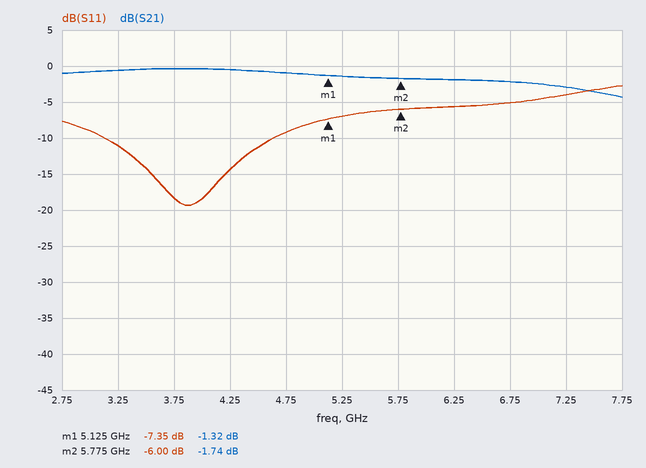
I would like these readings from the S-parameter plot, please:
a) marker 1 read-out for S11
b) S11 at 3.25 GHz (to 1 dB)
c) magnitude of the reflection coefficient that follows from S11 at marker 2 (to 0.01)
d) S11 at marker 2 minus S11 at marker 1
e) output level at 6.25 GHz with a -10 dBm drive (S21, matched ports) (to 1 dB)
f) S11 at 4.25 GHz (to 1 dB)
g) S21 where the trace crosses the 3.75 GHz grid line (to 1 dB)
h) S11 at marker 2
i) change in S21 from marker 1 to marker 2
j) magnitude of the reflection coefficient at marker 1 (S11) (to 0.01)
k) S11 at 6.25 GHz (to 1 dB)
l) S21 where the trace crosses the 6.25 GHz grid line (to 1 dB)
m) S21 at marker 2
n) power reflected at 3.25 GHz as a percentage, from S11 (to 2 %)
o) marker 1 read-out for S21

-7.35 dB
-11 dB
0.50
1.35 dB
-12 dBm
-14 dB
0 dB
-6.00 dB
-0.42 dB
0.43
-6 dB
-2 dB
-1.74 dB
8 %
-1.32 dB
